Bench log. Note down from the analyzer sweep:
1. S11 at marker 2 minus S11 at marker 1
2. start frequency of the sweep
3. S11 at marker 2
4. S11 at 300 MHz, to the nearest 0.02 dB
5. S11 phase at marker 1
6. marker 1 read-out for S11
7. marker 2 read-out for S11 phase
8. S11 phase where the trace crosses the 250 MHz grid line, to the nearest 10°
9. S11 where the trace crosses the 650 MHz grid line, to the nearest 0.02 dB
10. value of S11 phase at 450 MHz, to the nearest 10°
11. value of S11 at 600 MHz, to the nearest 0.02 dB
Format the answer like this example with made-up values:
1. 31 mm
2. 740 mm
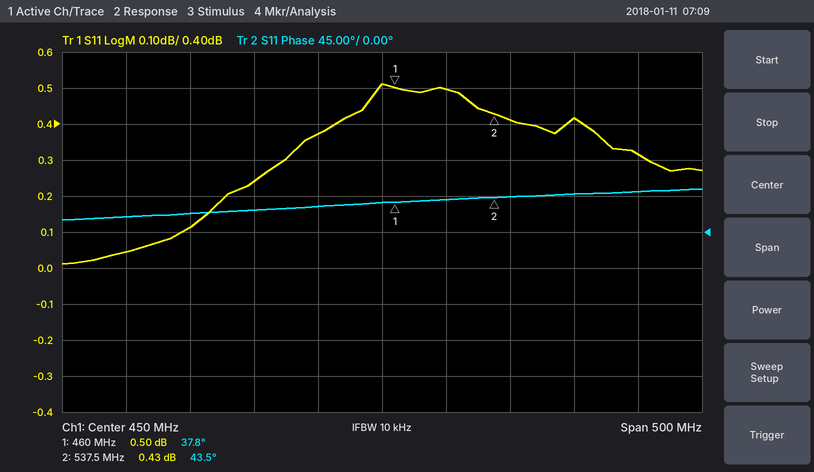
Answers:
1. -0.07 dB
2. 200 MHz
3. 0.43 dB
4. 0.12 dB
5. 37.8°
6. 0.50 dB
7. 43.5°
8. 20°
9. 0.32 dB
10. 40°
11. 0.42 dB
